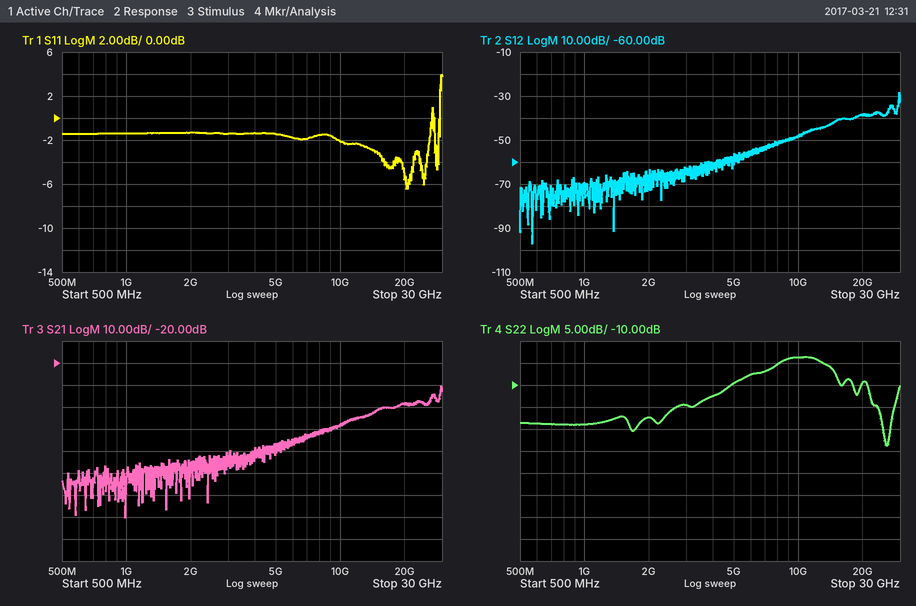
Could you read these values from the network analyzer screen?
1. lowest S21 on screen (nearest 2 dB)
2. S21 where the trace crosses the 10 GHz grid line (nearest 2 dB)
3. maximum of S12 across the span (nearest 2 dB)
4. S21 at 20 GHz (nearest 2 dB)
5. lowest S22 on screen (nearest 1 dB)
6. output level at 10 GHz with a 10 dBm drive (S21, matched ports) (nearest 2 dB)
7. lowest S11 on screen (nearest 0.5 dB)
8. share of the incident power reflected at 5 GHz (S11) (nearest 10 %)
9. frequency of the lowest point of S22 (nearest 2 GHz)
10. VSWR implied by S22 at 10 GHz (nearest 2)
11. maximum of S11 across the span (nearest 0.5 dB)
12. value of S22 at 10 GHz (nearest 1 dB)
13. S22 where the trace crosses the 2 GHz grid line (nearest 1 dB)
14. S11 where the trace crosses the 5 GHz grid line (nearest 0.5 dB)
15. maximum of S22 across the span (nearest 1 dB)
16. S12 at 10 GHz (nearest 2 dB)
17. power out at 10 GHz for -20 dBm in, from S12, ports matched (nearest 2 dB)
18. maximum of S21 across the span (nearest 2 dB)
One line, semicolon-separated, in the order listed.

-90 dB; -48 dB; -28 dB; -38 dB; -24 dB; -38 dBm; -6.5 dB; 70 %; 26 GHz; 4; 4.0 dB; -4 dB; -17 dB; -1.5 dB; -4 dB; -48 dB; -68 dBm; -30 dB
